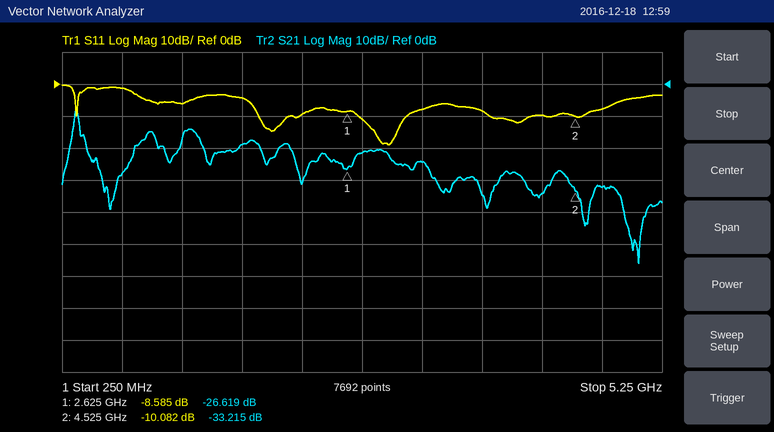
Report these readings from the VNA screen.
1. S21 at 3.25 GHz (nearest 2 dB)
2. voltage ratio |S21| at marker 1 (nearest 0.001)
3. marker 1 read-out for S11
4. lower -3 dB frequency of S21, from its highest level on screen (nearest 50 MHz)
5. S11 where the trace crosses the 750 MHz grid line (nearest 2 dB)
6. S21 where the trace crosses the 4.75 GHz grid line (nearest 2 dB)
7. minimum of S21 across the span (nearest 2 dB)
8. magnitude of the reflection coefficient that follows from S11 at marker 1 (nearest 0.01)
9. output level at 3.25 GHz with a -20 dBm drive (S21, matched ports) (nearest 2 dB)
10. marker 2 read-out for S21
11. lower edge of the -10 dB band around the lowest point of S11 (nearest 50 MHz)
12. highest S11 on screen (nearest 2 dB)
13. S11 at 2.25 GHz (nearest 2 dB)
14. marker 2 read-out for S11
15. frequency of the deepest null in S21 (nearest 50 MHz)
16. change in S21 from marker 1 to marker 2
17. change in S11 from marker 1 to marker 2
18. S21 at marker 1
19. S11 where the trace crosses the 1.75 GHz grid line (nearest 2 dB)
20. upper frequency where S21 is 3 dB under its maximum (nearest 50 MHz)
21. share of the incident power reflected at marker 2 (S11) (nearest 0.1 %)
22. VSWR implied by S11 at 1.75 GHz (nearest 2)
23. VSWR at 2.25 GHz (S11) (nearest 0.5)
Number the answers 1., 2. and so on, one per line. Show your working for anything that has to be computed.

1. -24 dB
2. 10^(-26.619/20) ≈ 0.047
3. -8.585 dB
4. 350 MHz
5. -2 dB
6. -32 dB
7. -56 dB
8. 10^(-8.585/20) ≈ 0.37
9. -20 dBm + (-24 dB) = -44 dBm
10. -33.215 dB
11. 2.70 GHz
12. 0 dB
13. -10 dB
14. -10.082 dB
15. 5.05 GHz
16. -33.215 − (-26.619) = -6.596 dB
17. -10.082 − (-8.585) = -1.497 dB
18. -26.619 dB
19. -4 dB
20. 400 MHz
21. 10^(-10.082/10) ≈ 9.8 %
22. |Γ| = 10^(-4/20) = 0.6310; VSWR = (1 + 0.6310)/(1 − 0.6310) ≈ 4
23. |Γ| = 10^(-10/20) = 0.3162; VSWR = (1 + 0.3162)/(1 − 0.3162) ≈ 1.92, so 2.0 to the nearest 0.5
